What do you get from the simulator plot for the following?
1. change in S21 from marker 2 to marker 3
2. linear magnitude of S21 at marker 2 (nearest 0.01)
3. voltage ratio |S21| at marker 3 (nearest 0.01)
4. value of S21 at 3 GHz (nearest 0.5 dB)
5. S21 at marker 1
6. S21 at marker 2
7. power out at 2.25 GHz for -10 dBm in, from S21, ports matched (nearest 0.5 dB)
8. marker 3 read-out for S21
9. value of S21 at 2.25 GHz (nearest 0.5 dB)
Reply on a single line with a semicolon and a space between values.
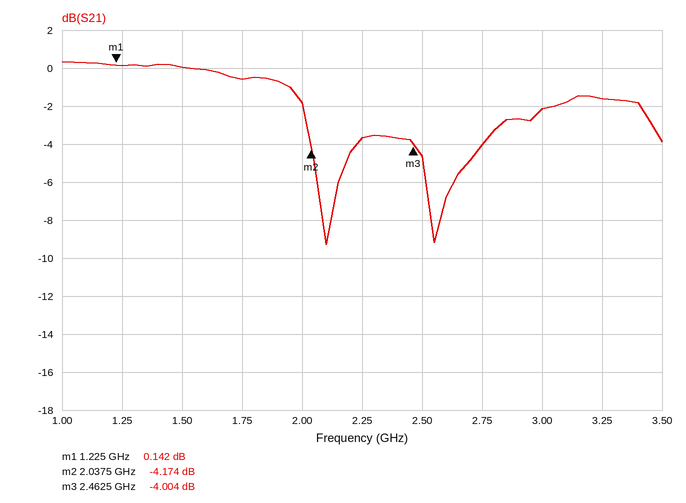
0.170 dB; 0.62; 0.63; -2.0 dB; 0.142 dB; -4.174 dB; -13.5 dBm; -4.004 dB; -3.5 dB
